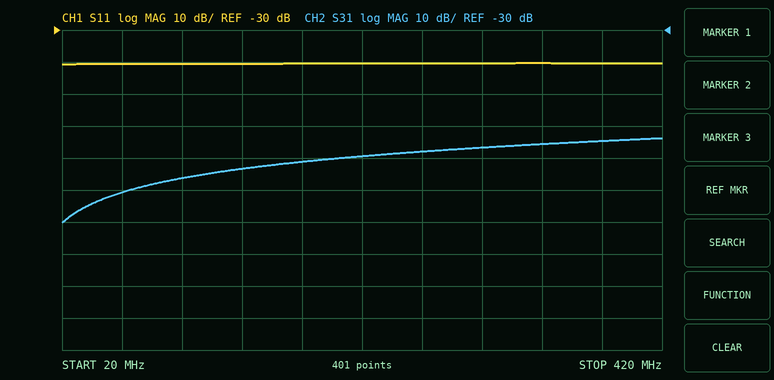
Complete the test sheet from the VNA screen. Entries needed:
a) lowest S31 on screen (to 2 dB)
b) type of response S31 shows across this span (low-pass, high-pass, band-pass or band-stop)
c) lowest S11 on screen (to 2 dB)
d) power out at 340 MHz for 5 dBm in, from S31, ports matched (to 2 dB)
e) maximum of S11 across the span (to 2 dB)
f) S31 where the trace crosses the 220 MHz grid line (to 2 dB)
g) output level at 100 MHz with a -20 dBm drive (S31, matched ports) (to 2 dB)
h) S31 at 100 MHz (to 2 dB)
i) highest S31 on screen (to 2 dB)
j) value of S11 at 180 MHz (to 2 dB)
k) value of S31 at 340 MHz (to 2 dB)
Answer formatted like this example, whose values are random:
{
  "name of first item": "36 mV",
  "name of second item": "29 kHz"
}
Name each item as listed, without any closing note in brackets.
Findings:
{
  "lowest S31 on screen": "-90 dB",
  "type of response S31 shows across this span": "high-pass",
  "lowest S11 on screen": "-40 dB",
  "power out at 340 MHz for 5 dBm in, from S31, ports matched": "-60 dBm",
  "maximum of S11 across the span": "-40 dB",
  "S31 where the trace crosses the 220 MHz grid line": "-70 dB",
  "output level at 100 MHz with a -20 dBm drive (S31, matched ports)": "-96 dBm",
  "S31 at 100 MHz": "-76 dB",
  "highest S31 on screen": "-64 dB",
  "value of S11 at 180 MHz": "-40 dB",
  "value of S31 at 340 MHz": "-66 dB"
}
